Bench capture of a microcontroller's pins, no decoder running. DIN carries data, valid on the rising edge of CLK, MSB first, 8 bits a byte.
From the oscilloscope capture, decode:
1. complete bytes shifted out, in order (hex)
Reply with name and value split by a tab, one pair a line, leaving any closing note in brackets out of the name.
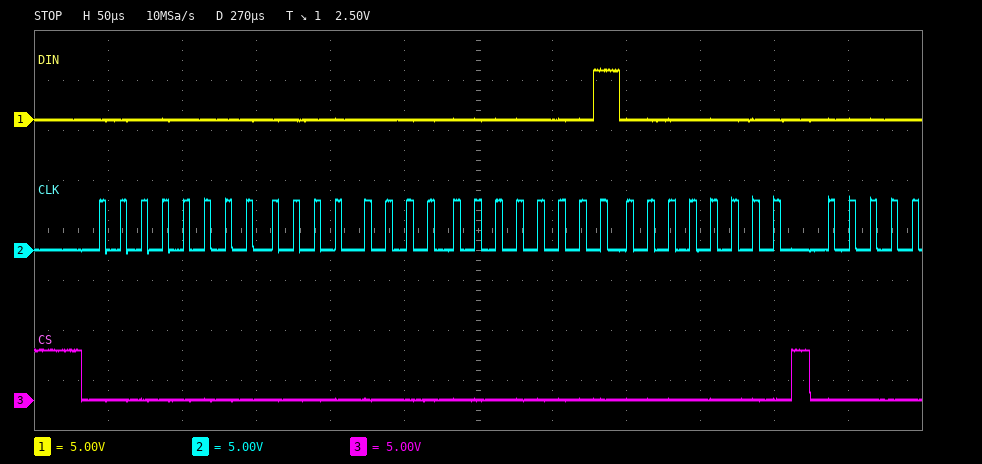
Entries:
complete bytes shifted out, in order	00 00 01 00
